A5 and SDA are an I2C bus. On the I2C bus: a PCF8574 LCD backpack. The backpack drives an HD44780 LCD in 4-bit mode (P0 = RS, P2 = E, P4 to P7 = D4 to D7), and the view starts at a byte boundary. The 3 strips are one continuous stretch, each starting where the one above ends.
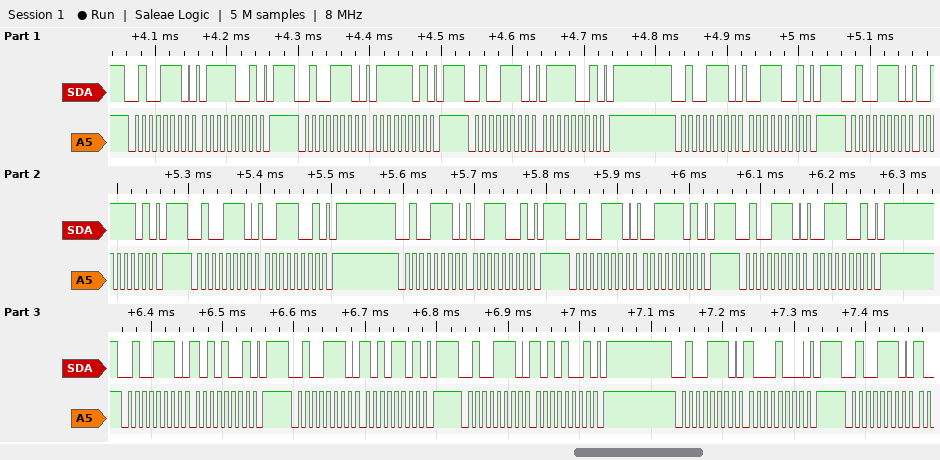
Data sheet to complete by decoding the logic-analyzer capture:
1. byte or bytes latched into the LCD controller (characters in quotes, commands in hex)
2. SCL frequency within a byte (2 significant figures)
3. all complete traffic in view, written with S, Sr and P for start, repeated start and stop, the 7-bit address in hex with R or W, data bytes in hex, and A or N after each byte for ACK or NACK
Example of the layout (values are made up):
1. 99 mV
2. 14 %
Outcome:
1. 's' ':'
2. 100 kHz
3. S 27W A 79 A P S 27W A 7D A P S 27W A 79 A P S 27W A 39 A P S 27W A 3D A P S 27W A 39 A P S 27W A 39 A P S 27W A 3D A P S 27W A 39 A P S 27W A A9 A P S 27W A AD A P S 27W A A9 A P S 27W A 88 A P S 27W A
